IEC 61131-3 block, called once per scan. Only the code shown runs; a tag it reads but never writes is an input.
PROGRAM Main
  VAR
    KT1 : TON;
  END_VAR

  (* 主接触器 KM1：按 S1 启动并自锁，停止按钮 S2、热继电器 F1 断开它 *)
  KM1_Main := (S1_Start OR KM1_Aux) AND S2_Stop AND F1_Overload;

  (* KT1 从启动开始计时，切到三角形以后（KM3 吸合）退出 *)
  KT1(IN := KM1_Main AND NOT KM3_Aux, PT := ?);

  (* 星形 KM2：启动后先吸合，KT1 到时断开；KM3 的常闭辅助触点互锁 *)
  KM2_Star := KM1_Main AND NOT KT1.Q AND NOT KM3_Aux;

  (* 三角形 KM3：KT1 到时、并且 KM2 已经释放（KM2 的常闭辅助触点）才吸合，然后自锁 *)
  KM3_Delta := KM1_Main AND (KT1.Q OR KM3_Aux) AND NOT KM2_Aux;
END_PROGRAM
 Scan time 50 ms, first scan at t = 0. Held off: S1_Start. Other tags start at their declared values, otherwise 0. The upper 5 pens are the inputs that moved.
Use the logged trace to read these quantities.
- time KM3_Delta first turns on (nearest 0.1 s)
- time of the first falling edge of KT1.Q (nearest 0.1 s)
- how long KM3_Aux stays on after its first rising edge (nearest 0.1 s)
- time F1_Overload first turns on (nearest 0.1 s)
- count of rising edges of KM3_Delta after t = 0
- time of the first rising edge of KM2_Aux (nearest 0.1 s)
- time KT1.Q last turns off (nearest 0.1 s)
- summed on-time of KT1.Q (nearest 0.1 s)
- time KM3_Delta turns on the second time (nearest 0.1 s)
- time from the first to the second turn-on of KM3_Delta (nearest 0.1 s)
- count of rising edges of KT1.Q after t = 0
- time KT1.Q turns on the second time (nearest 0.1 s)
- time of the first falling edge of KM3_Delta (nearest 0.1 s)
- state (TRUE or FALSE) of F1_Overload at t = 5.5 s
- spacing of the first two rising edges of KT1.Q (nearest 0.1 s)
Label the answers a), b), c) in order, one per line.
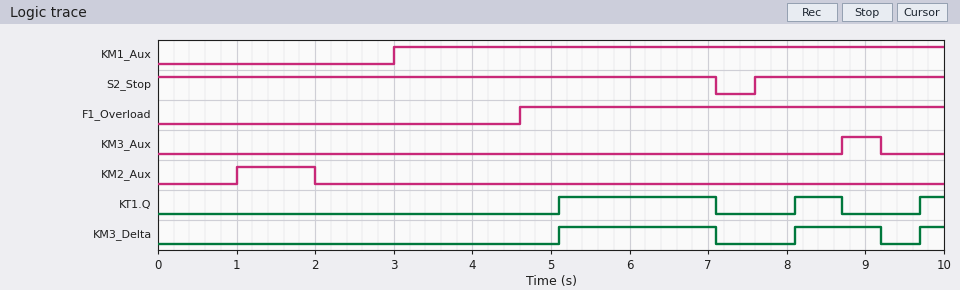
a) 5.1 s
b) 7.1 s
c) 0.5 s
d) 4.6 s
e) 3
f) 1.0 s
g) 8.7 s
h) 2.9 s
i) 8.1 s
j) 3.0 s
k) 3
l) 8.1 s
m) 7.1 s
n) TRUE
o) 3.0 s
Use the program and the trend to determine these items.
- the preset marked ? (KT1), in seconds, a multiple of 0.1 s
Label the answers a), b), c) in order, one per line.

a) 0.5 s
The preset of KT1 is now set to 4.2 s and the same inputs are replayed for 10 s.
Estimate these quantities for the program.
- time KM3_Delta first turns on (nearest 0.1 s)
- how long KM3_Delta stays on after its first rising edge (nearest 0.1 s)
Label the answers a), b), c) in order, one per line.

a) 8.7 s
b) 0.5 s
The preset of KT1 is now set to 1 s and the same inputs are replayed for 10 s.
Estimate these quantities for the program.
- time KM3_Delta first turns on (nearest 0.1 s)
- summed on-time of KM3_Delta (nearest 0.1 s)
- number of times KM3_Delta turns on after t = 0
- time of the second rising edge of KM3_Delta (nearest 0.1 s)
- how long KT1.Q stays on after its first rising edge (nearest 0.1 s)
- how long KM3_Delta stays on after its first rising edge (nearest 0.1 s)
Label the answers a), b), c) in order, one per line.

a) 5.6 s
b) 2.1 s
c) 2
d) 8.6 s
e) 1.5 s
f) 1.5 s
